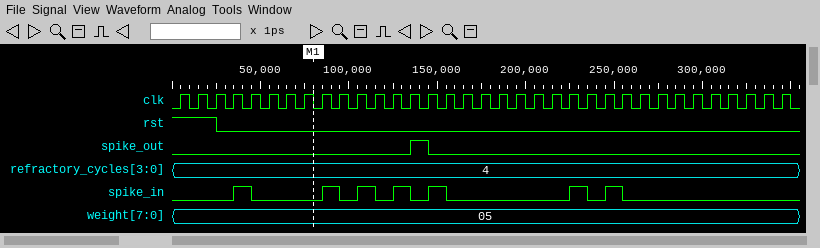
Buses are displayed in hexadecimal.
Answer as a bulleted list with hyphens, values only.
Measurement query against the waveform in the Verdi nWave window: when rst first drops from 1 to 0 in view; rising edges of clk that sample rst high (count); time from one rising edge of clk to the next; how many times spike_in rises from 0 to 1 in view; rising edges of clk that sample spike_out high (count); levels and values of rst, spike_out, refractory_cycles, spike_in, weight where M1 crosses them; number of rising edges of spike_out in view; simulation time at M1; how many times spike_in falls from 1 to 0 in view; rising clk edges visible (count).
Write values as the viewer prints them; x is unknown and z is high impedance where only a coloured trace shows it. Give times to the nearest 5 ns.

- 25 ns
- 3
- 10 ns
- 7
- 1
- rst=0, spike_out=0, refractory_cycles=4, spike_in=0, weight=05
- 1
- 80 ns
- 7
- 35
